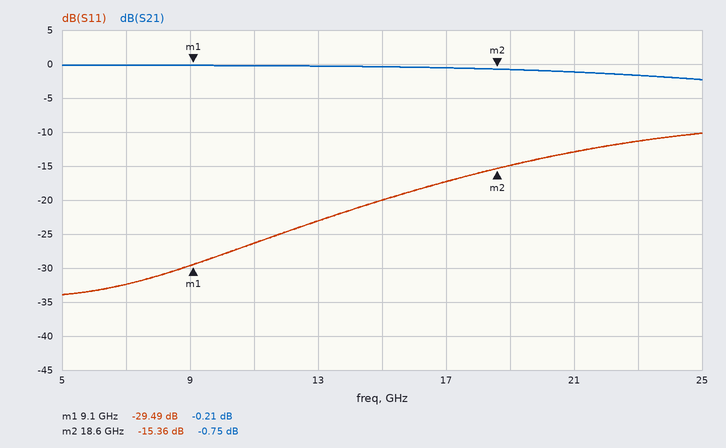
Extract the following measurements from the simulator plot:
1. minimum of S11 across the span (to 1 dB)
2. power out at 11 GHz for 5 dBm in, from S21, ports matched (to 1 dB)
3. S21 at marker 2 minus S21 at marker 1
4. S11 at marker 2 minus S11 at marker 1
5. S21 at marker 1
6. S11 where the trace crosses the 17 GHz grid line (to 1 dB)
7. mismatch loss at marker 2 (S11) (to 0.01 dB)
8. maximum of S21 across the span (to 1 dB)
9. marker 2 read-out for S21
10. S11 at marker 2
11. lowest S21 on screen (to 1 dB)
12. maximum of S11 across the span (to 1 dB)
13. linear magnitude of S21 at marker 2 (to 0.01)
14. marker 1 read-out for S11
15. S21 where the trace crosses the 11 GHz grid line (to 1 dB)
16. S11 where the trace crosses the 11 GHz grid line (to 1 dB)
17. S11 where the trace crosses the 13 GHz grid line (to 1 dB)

-34 dB
5 dBm
-0.54 dB
14.13 dB
-0.21 dB
-17 dB
0.13 dB
0 dB
-0.75 dB
-15.36 dB
-2 dB
-10 dB
0.92
-29.49 dB
0 dB
-26 dB
-23 dB
